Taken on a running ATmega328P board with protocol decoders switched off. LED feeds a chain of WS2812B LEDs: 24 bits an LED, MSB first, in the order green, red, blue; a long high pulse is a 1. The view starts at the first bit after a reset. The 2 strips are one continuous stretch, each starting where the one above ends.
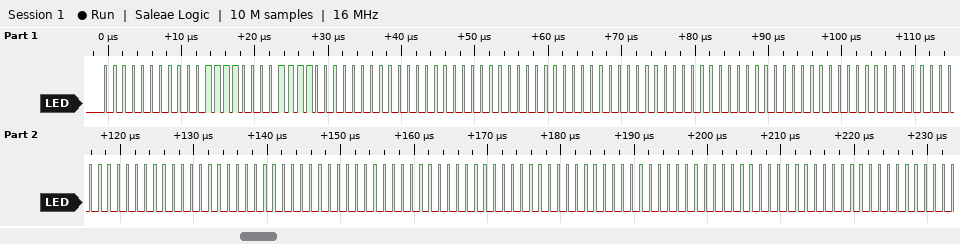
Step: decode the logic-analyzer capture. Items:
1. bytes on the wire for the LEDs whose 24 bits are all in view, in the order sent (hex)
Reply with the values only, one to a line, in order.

00 1E 1E 00 00 00 00 00 00 00 00 00 00 00 00 00 00 00 00 00 00
